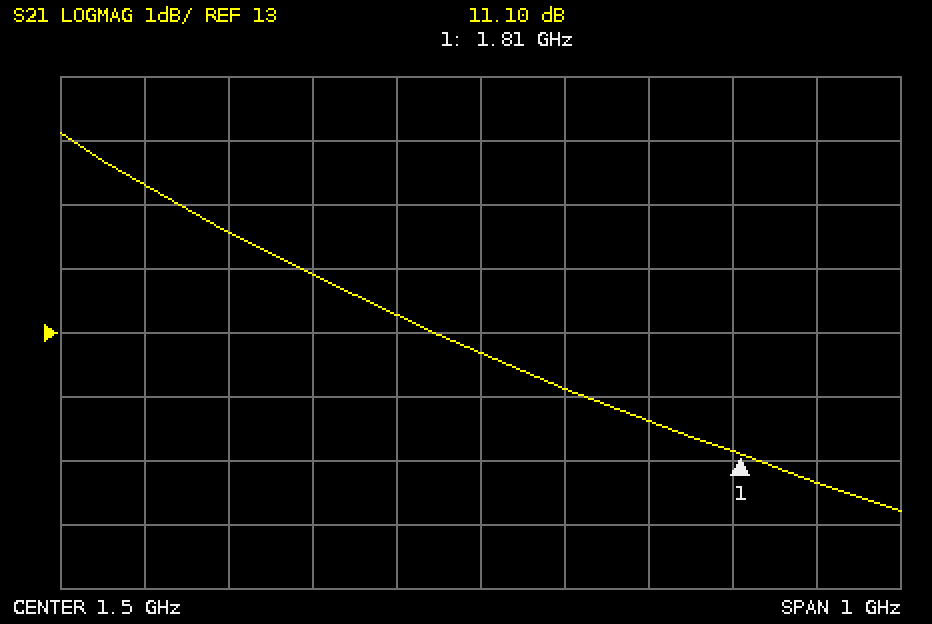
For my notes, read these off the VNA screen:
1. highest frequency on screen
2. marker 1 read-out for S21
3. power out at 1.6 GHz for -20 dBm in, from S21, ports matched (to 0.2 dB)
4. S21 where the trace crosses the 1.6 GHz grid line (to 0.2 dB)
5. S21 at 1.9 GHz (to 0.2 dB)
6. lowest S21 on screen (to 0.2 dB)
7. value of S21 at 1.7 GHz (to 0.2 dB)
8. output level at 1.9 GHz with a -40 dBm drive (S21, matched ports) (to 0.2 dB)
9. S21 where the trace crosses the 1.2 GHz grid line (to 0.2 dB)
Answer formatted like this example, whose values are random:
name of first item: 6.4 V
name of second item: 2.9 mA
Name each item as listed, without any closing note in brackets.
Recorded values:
highest frequency on screen: 2 GHz
marker 1 read-out for S21: 11.10 dB
power out at 1.6 GHz for -20 dBm in, from S21, ports matched: -7.8 dBm
S21 where the trace crosses the 1.6 GHz grid line: 12.2 dB
S21 at 1.9 GHz: 10.6 dB
lowest S21 on screen: 10.2 dB
value of S21 at 1.7 GHz: 11.6 dB
output level at 1.9 GHz with a -40 dBm drive (S21, matched ports): -29.4 dBm
S21 where the trace crosses the 1.2 GHz grid line: 14.6 dB
